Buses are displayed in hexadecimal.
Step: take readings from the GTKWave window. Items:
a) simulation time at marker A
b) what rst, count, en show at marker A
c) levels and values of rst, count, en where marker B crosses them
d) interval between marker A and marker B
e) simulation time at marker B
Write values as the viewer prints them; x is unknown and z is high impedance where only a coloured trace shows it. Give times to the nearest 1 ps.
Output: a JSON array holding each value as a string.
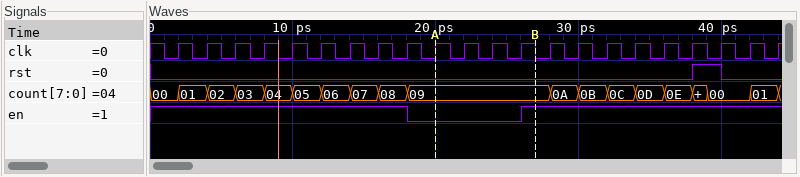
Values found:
["20 ps", "rst=0, count=09, en=0", "rst=0, count=09, en=1", "7 ps", "27 ps"]
